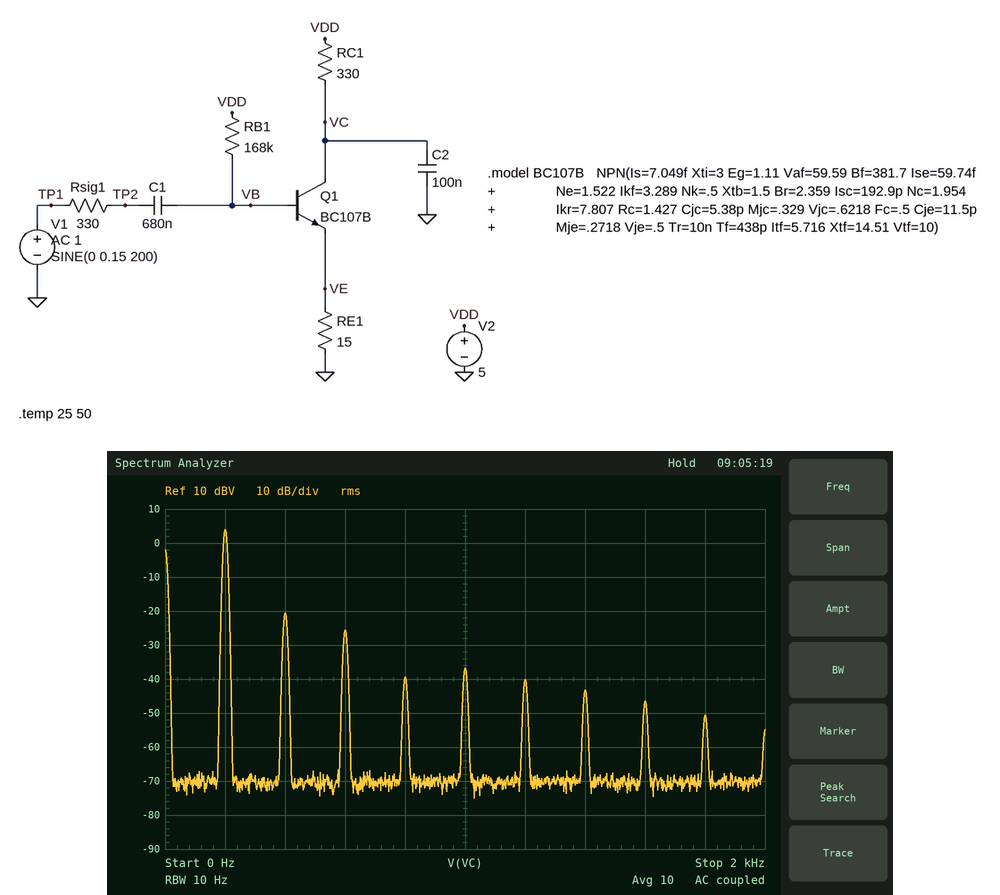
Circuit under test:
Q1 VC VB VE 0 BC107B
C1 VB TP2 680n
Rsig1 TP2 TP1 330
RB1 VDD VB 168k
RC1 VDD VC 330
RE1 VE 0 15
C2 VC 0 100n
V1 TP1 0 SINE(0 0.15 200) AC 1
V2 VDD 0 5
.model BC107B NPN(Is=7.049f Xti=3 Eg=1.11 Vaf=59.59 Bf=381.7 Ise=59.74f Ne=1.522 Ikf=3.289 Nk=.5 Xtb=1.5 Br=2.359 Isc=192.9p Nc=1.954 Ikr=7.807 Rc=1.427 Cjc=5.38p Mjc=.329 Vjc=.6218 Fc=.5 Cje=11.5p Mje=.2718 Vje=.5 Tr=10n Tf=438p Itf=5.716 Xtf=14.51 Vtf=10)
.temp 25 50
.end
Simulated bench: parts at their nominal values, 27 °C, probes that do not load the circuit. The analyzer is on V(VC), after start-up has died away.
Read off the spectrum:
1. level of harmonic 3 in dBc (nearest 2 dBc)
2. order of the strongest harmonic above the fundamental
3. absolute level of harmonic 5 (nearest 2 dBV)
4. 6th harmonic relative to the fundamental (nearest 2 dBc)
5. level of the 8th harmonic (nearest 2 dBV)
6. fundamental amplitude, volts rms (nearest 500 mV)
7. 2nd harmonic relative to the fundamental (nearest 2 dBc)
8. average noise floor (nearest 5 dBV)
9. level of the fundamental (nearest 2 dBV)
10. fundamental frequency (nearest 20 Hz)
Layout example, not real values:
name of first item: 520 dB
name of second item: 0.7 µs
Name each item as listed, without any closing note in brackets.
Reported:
level of harmonic 3 in dBc: -30 dBc
order of the strongest harmonic above the fundamental: 2
absolute level of harmonic 5: -36 dBV
6th harmonic relative to the fundamental: -44 dBc
level of the 8th harmonic: -46 dBV
fundamental amplitude, volts rms: 1.5 V
2nd harmonic relative to the fundamental: -24 dBc
average noise floor: -70 dBV
level of the fundamental: 4 dBV
fundamental frequency: 200 Hz
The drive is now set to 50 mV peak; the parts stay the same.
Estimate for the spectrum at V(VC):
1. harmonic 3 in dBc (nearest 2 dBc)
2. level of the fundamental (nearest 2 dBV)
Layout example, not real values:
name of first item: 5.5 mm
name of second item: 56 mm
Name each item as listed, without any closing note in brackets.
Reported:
harmonic 3 in dBc: -58 dBc
level of the fundamental: -4 dBV
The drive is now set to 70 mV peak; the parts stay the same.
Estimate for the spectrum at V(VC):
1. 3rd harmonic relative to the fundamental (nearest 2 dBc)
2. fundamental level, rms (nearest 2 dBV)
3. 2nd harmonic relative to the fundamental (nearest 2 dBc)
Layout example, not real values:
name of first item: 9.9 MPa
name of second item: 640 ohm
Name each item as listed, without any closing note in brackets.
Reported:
3rd harmonic relative to the fundamental: -52 dBc
fundamental level, rms: -2 dBV
2nd harmonic relative to the fundamental: -34 dBc
